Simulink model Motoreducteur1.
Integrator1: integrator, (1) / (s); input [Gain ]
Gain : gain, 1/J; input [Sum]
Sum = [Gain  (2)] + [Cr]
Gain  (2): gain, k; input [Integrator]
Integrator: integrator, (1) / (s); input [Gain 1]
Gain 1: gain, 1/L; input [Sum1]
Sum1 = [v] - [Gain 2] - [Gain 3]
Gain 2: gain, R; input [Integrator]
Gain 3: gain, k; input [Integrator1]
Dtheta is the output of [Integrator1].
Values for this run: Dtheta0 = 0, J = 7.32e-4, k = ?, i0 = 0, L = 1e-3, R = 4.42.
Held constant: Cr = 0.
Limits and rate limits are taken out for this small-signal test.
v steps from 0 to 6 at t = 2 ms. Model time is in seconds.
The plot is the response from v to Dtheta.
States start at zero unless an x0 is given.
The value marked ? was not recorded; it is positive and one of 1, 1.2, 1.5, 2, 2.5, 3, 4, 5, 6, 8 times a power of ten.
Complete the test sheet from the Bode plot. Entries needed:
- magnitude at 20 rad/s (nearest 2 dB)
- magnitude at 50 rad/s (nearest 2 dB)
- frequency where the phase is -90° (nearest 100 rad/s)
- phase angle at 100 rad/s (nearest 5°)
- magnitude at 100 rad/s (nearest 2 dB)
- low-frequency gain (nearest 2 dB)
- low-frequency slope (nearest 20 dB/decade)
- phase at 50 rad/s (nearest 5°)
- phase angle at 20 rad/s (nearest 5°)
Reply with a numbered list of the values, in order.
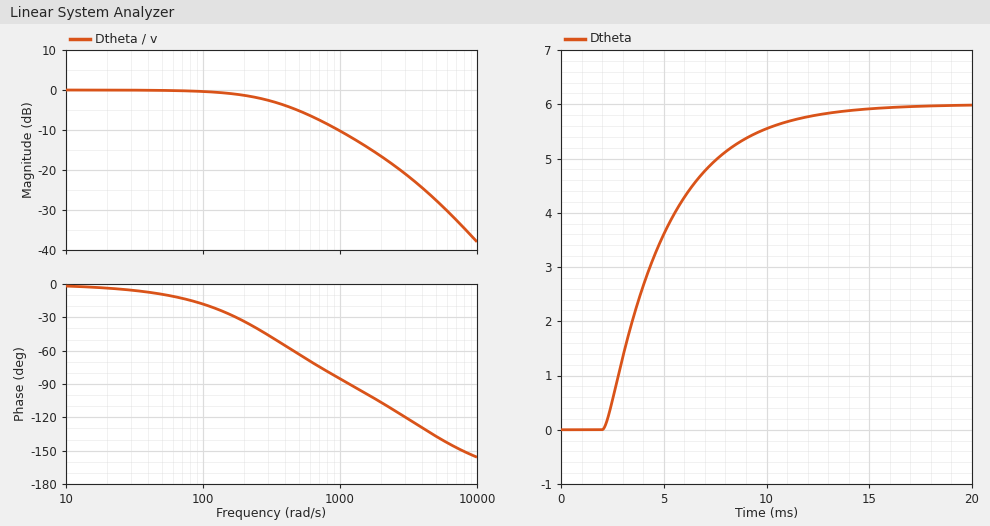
1. 0 dB
2. 0 dB
3. 1200 rad/s
4. -20°
5. 0 dB
6. 0 dB
7. 0 dB/decade
8. -10°
9. -5°
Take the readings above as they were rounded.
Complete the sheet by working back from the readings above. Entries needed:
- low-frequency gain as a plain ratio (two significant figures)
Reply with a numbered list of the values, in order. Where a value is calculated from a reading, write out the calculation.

1. 10^(0 / 20) = 1.0
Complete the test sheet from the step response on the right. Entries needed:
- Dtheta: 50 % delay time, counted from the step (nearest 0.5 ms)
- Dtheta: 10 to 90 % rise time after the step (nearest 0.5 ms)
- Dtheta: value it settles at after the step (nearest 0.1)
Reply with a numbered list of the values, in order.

1. 2.5 ms
2. 6.5 ms
3. 6.0
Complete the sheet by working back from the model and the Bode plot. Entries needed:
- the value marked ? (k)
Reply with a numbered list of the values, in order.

1. 1
